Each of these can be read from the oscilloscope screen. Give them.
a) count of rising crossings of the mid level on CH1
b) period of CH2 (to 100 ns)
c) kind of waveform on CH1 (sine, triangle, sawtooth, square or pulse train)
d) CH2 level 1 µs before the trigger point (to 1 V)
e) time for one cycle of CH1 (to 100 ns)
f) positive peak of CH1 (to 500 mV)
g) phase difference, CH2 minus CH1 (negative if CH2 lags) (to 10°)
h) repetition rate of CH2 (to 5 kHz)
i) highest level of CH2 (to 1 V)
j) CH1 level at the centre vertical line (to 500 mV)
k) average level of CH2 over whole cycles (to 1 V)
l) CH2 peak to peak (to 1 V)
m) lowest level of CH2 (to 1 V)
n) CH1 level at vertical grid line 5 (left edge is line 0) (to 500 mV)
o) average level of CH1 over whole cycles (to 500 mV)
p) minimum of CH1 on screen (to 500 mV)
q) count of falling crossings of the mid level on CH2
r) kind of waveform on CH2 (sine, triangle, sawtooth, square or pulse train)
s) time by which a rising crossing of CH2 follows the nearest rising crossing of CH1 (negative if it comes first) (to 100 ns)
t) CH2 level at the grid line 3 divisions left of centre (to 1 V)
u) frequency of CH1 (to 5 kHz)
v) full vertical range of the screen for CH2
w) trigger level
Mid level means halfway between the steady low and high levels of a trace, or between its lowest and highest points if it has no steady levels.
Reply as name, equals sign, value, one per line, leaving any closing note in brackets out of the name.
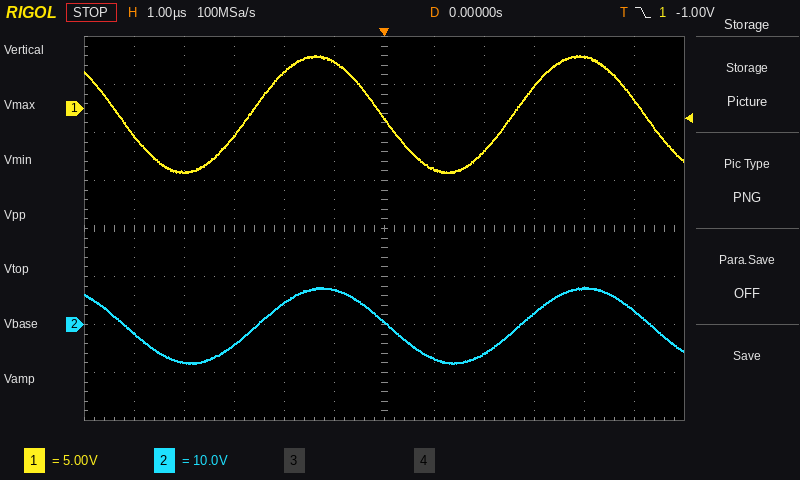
count of rising crossings of the mid level on CH1 = 2
period of CH2 = 5.3 µs
kind of waveform on CH1 = sine
CH2 level 1 µs before the trigger point = 7 V
time for one cycle of CH1 = 5.3 µs
positive peak of CH1 = 5.5 V
phase difference, CH2 minus CH1 (negative if CH2 lags) = -10°
repetition rate of CH2 = 190 kHz
highest level of CH2 = 8 V
CH1 level at the centre vertical line = -1.0 V
average level of CH2 over whole cycles = 0 V
CH2 peak to peak = 16 V
lowest level of CH2 = -8 V
CH1 level at vertical grid line 5 (left edge is line 0) = 5.0 V
average level of CH1 over whole cycles = -500 mV
minimum of CH1 on screen = -6.5 V
count of falling crossings of the mid level on CH2 = 3
kind of waveform on CH2 = sine
time by which a rising crossing of CH2 follows the nearest rising crossing of CH1 (negative if it comes first) = +100 ns
CH2 level at the grid line 3 divisions left of centre = -4 V
frequency of CH1 = 190 kHz
full vertical range of the screen for CH2 = 80 V
trigger level = -1.00 V
